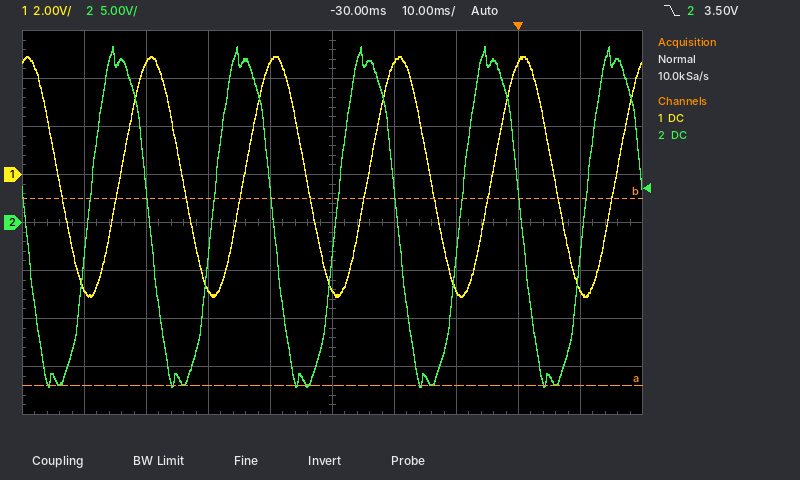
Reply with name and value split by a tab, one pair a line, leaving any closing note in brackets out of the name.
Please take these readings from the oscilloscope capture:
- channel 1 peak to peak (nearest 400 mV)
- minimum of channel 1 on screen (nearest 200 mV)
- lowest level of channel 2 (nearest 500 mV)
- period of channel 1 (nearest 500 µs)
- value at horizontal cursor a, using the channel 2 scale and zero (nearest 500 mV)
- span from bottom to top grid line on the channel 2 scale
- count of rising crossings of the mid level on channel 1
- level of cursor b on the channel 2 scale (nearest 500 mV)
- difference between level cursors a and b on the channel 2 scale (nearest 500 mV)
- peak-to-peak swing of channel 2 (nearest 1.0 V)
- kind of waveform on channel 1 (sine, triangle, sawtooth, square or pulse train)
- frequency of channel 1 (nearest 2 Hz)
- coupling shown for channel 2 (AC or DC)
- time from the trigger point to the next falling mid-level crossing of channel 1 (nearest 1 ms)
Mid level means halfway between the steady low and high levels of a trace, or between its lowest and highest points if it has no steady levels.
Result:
channel 1 peak to peak	10.0 V
minimum of channel 1 on screen	-5.0 V
lowest level of channel 2	-17.0 V
period of channel 1	20.0 ms
value at horizontal cursor a, using the channel 2 scale and zero	-17.0 V
span from bottom to top grid line on the channel 2 scale	40 V
count of rising crossings of the mid level on channel 1	5
level of cursor b on the channel 2 scale	2.5 V
difference between level cursors a and b on the channel 2 scale	19.5 V
peak-to-peak swing of channel 2	35.0 V
kind of waveform on channel 1	sine
frequency of channel 1	50 Hz
coupling shown for channel 2	DC
time from the trigger point to the next falling mid-level crossing of channel 1	6 ms
